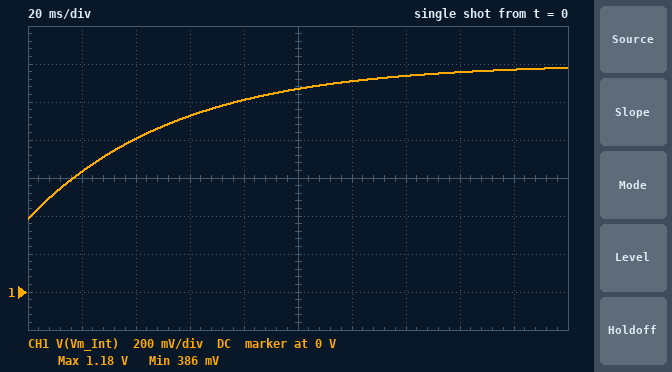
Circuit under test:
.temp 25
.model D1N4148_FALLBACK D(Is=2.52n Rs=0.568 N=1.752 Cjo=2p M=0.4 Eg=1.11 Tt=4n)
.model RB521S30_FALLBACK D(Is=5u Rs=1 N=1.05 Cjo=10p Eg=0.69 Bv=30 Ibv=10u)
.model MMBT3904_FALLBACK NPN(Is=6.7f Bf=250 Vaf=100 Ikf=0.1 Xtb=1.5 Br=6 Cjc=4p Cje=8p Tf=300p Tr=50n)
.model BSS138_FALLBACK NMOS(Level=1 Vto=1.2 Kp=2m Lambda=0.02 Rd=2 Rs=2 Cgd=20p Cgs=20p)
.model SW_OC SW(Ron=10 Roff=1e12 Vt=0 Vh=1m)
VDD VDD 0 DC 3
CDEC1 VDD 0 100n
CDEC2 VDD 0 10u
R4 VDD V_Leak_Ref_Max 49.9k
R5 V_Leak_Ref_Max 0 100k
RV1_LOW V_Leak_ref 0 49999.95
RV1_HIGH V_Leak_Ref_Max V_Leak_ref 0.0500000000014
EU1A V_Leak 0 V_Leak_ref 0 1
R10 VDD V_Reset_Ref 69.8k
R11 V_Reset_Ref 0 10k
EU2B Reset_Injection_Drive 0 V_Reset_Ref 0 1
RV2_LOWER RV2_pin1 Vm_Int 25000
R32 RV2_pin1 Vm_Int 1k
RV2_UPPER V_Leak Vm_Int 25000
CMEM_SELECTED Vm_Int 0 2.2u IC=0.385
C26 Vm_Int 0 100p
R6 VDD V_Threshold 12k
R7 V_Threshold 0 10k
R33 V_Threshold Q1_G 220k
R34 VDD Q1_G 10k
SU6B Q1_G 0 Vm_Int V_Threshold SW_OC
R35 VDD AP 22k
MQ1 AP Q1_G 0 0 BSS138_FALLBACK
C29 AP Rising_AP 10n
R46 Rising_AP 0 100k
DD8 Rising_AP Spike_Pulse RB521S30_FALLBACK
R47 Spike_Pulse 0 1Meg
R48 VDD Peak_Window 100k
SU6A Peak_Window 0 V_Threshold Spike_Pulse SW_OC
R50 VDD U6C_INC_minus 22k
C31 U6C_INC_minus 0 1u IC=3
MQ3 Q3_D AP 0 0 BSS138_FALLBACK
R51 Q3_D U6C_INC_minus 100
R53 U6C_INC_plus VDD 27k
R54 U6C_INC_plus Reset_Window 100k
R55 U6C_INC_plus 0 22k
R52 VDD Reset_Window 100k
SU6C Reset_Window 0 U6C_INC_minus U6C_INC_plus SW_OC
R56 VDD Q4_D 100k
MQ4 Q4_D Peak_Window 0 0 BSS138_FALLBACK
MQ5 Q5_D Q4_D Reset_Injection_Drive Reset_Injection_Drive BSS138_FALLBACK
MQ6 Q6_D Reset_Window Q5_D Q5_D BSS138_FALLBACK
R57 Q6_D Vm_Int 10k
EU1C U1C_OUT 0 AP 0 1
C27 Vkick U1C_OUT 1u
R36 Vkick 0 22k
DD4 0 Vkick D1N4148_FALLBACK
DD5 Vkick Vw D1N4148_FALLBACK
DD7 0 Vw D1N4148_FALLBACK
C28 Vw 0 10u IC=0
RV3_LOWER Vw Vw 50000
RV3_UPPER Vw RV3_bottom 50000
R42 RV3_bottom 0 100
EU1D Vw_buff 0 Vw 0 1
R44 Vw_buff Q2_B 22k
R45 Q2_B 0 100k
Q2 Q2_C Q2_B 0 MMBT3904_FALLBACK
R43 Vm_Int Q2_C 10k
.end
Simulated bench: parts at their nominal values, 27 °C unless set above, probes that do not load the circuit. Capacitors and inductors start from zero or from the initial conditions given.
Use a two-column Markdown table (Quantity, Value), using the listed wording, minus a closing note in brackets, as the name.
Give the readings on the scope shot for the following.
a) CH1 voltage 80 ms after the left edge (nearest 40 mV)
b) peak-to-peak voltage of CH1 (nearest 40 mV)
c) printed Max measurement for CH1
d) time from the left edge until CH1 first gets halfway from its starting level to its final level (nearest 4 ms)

| Quantity | Value |
|---|---|
| CH1 voltage 80 ms after the left edge | 1.00 V |
| peak-to-peak voltage of CH1 | 800 mV |
| printed Max measurement for CH1 | 1.18 V |
| time from the left edge until CH1 first gets halfway from its starting level to its final level | 36 ms |
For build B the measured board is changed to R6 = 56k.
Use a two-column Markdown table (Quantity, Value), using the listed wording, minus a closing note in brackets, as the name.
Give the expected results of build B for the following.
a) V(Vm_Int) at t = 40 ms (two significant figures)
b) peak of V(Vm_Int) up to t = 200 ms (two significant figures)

| Quantity | Value |
|---|---|
| V(Vm_Int) at t = 40 ms | 620 mV |
| peak of V(Vm_Int) up to t = 200 ms | 630 mV |
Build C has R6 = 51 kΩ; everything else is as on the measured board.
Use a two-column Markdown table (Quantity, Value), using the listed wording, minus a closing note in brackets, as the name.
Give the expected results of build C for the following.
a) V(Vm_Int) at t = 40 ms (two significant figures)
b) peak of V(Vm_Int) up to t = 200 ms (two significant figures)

| Quantity | Value |
|---|---|
| V(Vm_Int) at t = 40 ms | 620 mV |
| peak of V(Vm_Int) up to t = 200 ms | 630 mV |
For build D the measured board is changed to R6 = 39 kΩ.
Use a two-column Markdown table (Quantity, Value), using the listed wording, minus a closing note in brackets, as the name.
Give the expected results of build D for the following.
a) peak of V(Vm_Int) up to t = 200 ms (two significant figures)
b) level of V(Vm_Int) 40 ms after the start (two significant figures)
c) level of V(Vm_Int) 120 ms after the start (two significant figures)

| Quantity | Value |
|---|---|
| peak of V(Vm_Int) up to t = 200 ms | 710 mV |
| level of V(Vm_Int) 40 ms after the start | 670 mV |
| level of V(Vm_Int) 120 ms after the start | 630 mV |
